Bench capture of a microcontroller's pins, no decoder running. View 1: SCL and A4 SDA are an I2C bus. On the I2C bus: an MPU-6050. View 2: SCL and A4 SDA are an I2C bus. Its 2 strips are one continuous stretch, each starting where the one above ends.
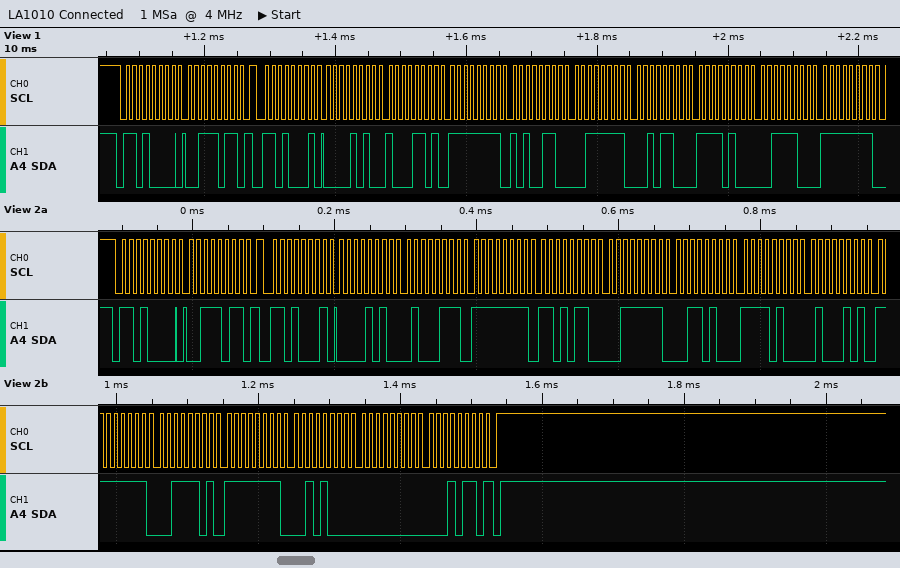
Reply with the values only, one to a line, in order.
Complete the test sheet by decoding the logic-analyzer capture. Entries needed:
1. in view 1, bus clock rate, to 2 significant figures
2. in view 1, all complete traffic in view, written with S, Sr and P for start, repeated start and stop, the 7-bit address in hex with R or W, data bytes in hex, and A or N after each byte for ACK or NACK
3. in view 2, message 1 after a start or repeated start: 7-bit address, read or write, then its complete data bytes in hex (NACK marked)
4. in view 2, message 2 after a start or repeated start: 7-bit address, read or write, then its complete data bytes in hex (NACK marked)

100 kHz
S 68W A 3B A Sr 68R A 0A A 8D A FF A A6 A 3F A 2C A F4 A 3C A FF A
0x68 write: 3B
0x68 read: 0A 47 FF D6 3F 34 F4 45 FF 3D FF 28 00 16 NACK
